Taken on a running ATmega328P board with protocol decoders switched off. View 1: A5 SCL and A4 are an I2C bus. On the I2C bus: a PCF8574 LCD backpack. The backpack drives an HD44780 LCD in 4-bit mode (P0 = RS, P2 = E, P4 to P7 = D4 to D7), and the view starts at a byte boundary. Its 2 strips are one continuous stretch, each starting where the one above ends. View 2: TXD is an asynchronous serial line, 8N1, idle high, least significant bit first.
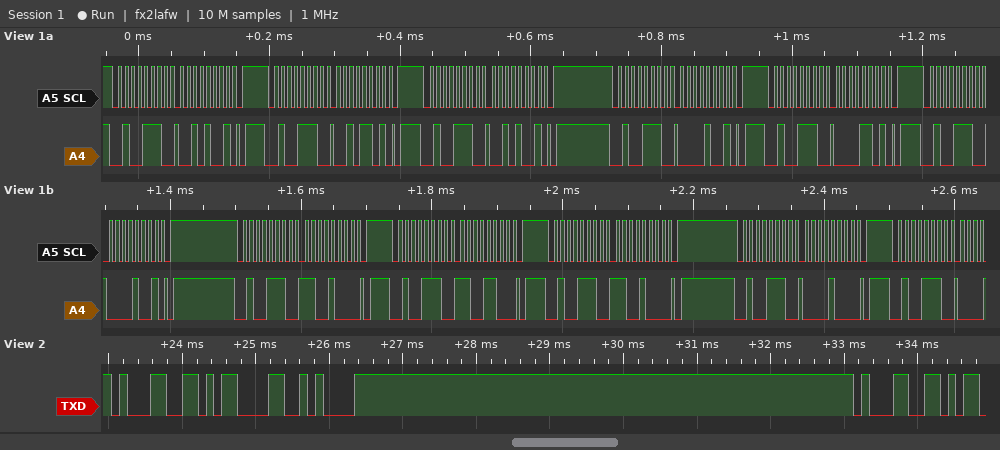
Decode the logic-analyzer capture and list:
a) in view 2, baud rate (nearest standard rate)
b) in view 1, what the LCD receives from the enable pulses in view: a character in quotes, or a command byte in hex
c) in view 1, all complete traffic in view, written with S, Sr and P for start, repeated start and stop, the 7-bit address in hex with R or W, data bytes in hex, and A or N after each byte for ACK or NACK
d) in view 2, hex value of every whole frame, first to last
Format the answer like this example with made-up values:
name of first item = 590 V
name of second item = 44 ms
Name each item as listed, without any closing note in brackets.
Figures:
in view 2, baud rate = 9600 baud
in view 1, what the LCD receives from the enable pulses in view: a character in quotes, or a command byte in hex = ' '
in view 1, all complete traffic in view, written with S, Sr and P for start, repeated start and stop, the 7-bit address in hex with R or W, data bytes in hex, and A or N after each byte for ACK or NACK = S 27W A 29 A P S 27W A 2D A P S 27W A 29 A P S 27W A 09 A P S 27W A 0D A P S 27W A 09 A P S 27W A C8 A P S 27W A CC A P S 27W A C8 A P S 27W A 08 A P S 27W A
in view 2, hex value of every whole frame, first to last = 31 0D 0A 31
